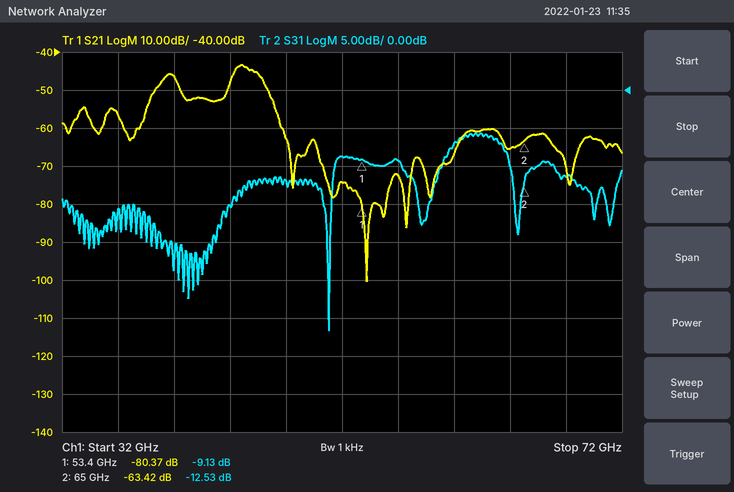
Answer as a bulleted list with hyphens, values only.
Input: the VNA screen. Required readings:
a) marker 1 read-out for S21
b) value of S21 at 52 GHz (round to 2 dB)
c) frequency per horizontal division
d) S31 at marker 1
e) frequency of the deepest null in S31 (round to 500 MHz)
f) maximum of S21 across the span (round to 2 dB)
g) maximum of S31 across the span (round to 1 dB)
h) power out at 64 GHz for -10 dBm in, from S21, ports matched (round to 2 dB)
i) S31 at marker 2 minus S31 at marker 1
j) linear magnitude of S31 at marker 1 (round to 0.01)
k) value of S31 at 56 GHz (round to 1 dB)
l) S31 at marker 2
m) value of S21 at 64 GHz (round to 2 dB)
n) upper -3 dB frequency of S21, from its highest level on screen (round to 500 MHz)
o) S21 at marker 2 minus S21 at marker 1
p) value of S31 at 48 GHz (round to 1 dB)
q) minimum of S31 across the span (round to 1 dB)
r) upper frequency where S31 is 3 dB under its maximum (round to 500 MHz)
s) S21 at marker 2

- -80.37 dB
- -74 dB
- 4 GHz
- -9.13 dB
- 51.0 GHz
- -44 dB
- -6 dB
- -76 dBm
- -3.40 dB
- 0.35
- -9 dB
- -12.53 dB
- -66 dB
- 46.0 GHz
- 16.95 dB
- -12 dB
- -32 dB
- 64.0 GHz
- -63.42 dB
